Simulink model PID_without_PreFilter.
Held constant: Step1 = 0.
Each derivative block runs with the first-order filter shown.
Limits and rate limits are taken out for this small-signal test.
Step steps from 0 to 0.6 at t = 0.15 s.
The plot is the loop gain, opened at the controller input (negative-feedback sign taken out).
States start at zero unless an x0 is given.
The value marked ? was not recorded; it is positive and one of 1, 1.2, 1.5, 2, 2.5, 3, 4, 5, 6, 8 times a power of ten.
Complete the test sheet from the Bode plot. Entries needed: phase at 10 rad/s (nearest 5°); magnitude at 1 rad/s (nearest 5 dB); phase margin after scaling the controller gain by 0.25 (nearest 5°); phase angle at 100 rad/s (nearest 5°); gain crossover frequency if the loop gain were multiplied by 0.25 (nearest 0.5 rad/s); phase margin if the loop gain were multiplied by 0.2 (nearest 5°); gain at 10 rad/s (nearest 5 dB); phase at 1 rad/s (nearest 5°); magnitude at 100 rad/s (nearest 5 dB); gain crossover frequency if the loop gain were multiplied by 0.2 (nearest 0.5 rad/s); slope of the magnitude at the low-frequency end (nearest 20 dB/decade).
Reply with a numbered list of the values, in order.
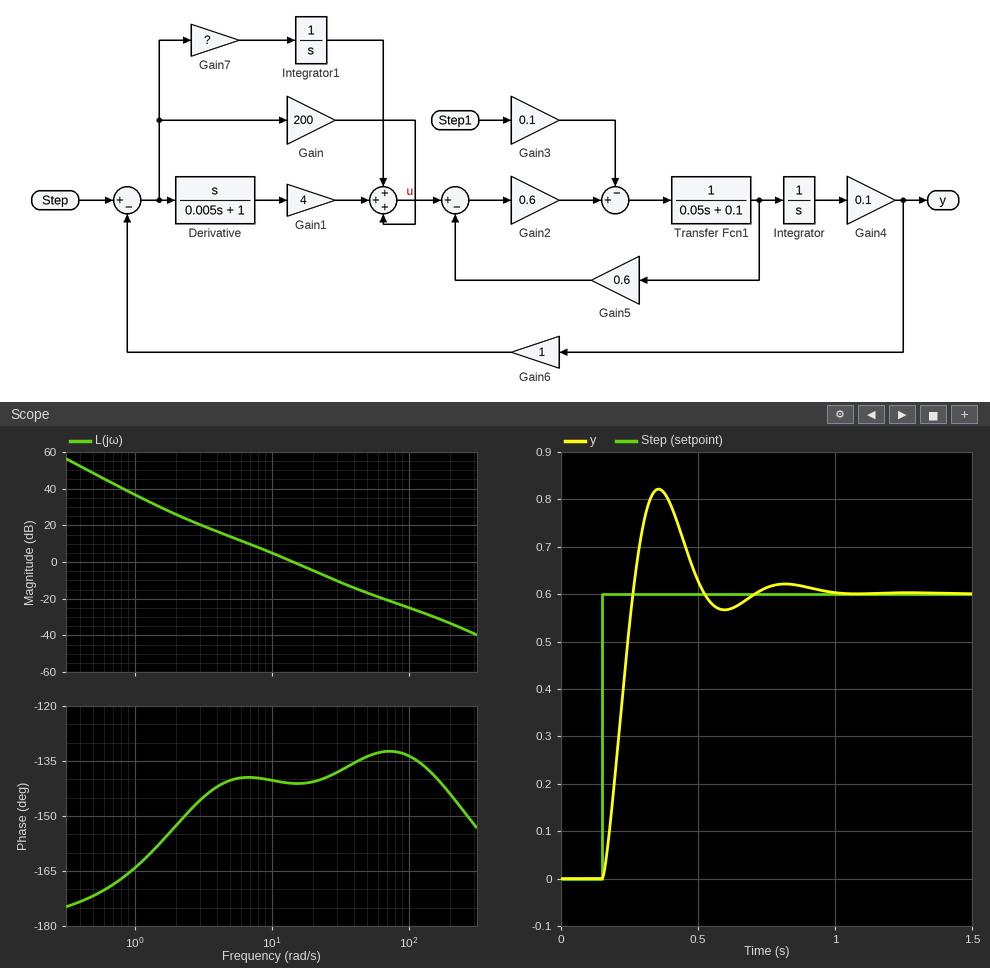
1. -140°
2. 35 dB
3. 40°
4. -135°
5. 6.0 rad/s
6. 40°
7. 5 dB
8. -165°
9. -25 dB
10. 5.0 rad/s
11. -40 dB/decade
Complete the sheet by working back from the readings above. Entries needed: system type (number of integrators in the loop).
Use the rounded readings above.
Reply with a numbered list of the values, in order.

1. 2
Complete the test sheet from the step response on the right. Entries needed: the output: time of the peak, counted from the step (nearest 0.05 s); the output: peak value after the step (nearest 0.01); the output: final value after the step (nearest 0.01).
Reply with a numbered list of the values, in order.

1. 0.20 s
2. 0.82
3. 0.60
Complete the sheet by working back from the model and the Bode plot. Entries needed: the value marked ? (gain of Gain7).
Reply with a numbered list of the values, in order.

1. 500
